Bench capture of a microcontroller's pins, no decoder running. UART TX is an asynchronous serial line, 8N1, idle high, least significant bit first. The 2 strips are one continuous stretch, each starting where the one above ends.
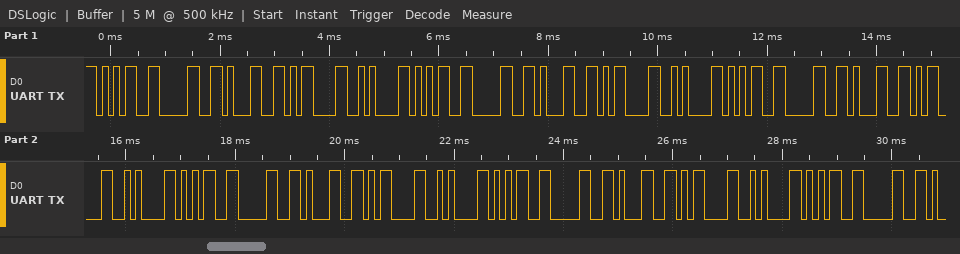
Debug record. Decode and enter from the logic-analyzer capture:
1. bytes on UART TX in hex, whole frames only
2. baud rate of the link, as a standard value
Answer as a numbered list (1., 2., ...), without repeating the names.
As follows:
1. 35 30 31 0D 0A 35 30 31 0D 0A 35 30 31 0D 0A 35 30 31 0D 0A 35 30 31 0D 0A 35 30
2. 9600 baud
